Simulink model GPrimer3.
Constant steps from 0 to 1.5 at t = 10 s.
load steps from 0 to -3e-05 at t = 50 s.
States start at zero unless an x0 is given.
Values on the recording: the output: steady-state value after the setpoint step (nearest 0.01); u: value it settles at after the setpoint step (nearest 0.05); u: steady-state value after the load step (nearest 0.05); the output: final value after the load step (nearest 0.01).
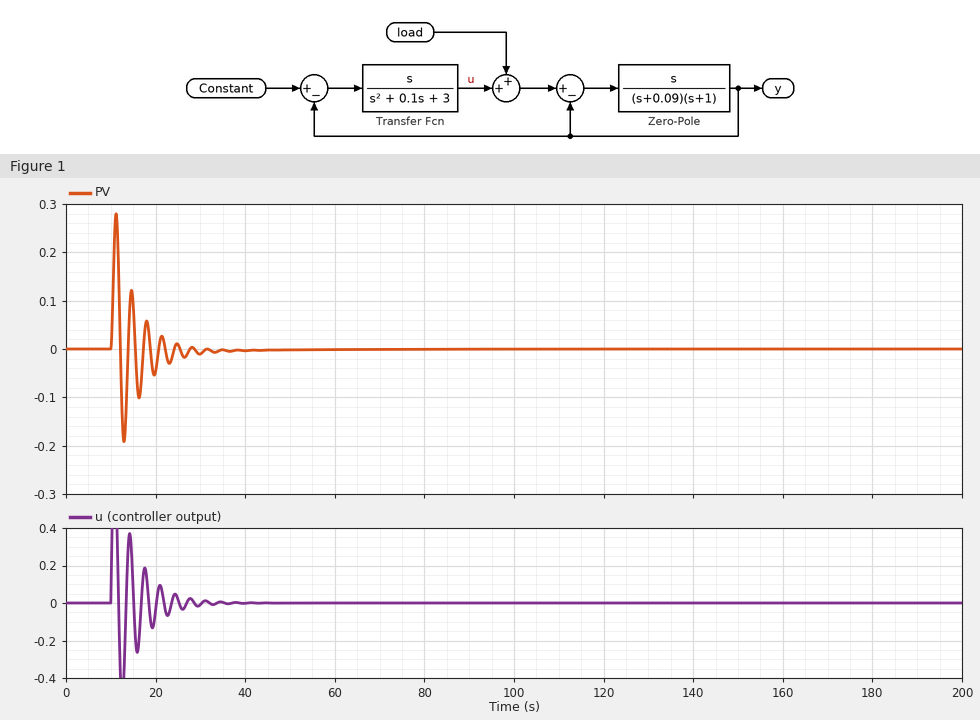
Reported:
0.00
0.00
0.00
0.00
